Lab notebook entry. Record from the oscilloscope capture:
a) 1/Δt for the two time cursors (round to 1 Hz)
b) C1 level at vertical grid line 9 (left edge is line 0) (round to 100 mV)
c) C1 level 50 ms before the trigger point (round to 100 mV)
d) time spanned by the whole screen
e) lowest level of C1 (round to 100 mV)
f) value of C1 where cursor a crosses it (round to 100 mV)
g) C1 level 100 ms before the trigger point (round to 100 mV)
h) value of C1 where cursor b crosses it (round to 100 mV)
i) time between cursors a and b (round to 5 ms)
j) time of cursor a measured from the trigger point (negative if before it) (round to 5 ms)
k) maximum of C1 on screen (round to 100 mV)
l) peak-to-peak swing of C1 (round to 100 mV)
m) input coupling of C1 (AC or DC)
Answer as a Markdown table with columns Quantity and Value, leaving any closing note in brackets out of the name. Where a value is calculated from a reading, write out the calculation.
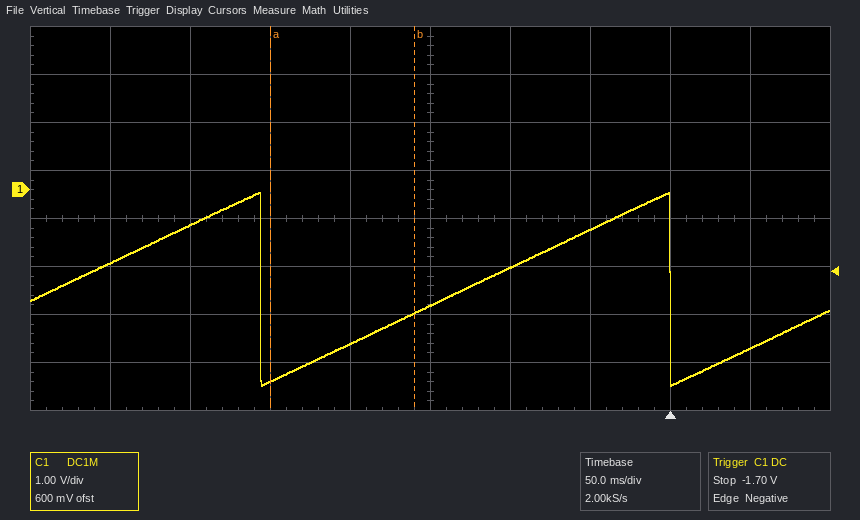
| Quantity | Value |
|---|---|
| 1/Δt for the two time cursors | 1 / 90 ms ≈ 11 Hz |
| C1 level at vertical grid line 9 (left edge is line 0) | -3.3 V |
| C1 level 50 ms before the trigger point | -800 mV |
| time spanned by the whole screen | 500 ms |
| lowest level of C1 | -4.1 V |
| value of C1 where cursor a crosses it | -4.0 V |
| C1 level 100 ms before the trigger point | -1.6 V |
| value of C1 where cursor b crosses it | -2.6 V |
| time between cursors a and b | 90 ms |
| time of cursor a measured from the trigger point (negative if before it) | -250 ms |
| maximum of C1 on screen | -100 mV |
| peak-to-peak swing of C1 | -100 mV − (-4.1 V) = 4.0 V |
| input coupling of C1 | DC |
